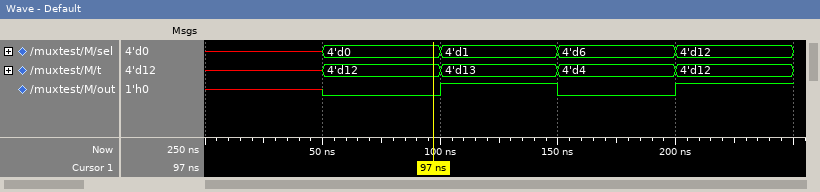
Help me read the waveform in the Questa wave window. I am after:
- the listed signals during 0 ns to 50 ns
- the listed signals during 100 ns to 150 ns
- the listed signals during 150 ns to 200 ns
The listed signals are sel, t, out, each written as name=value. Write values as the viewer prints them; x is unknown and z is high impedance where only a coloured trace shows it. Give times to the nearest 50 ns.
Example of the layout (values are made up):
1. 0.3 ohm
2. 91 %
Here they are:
1. sel=x, t=x, out=x
2. sel=4'd1, t=4'd13, out=1
3. sel=4'd6, t=4'd4, out=0
